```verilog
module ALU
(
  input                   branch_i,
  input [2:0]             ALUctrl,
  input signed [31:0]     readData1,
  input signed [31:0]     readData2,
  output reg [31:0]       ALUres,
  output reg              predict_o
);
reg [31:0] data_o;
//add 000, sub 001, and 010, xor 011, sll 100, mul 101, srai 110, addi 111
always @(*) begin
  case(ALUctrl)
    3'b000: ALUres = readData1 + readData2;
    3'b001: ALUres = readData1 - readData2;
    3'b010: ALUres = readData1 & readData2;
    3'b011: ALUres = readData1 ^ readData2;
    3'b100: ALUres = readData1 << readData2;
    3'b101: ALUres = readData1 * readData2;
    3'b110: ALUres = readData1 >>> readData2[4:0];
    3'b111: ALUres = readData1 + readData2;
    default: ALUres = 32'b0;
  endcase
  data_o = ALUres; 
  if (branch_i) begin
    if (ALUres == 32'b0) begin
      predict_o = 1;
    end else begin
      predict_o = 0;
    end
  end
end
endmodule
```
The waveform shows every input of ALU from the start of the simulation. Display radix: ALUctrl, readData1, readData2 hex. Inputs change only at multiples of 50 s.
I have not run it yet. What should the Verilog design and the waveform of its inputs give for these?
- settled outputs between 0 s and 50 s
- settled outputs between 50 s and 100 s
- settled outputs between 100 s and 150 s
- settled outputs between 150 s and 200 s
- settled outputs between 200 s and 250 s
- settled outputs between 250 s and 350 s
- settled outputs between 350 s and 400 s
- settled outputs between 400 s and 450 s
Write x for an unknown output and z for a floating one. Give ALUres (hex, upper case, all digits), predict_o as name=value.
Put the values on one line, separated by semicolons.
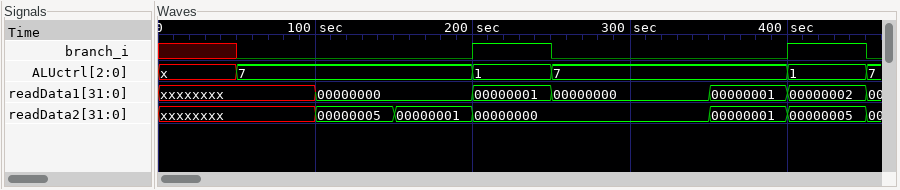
ALUres=x, predict_o=x; ALUres=x, predict_o=x; ALUres=00000005, predict_o=x; ALUres=00000001, predict_o=x; ALUres=00000001, predict_o=0; ALUres=00000000, predict_o=0; ALUres=00000002, predict_o=0; ALUres=FFFFFFFD, predict_o=0
